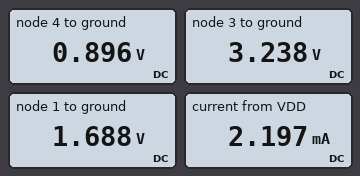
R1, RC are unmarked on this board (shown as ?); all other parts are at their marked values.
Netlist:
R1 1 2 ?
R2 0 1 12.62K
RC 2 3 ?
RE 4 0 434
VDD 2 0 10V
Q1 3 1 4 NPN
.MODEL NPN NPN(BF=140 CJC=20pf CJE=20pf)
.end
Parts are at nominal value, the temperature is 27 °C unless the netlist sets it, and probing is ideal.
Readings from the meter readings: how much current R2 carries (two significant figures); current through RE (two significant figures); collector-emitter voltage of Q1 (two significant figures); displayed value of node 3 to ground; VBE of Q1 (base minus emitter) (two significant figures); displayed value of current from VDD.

130 µA
2.1 mA
2.3 V
3.238 V
790 mV
2.197 mA
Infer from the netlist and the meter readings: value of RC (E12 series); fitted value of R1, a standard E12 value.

3.3 kΩ
56 kΩ
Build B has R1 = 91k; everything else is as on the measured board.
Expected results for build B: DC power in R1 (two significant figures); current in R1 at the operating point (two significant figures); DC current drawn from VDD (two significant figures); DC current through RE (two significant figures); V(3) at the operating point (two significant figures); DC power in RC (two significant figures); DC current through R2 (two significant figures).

860 µW
97 µA
960 µA
870 µA
7.1 V
2.5 mW
91 µA
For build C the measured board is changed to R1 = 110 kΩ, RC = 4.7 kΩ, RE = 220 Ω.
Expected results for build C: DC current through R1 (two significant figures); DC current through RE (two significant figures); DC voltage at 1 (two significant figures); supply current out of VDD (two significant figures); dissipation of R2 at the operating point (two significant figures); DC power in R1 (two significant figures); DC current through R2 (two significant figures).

82 µA
860 µA
960 mV
940 µA
73 µW
740 µW
76 µA
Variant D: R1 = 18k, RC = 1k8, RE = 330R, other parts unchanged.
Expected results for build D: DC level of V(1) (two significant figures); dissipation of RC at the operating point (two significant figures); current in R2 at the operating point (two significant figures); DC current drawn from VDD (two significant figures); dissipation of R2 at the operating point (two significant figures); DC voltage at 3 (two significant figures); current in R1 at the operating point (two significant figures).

2.4 V
38 mW
190 µA
5.0 mA
460 µW
1.7 V
420 µA
